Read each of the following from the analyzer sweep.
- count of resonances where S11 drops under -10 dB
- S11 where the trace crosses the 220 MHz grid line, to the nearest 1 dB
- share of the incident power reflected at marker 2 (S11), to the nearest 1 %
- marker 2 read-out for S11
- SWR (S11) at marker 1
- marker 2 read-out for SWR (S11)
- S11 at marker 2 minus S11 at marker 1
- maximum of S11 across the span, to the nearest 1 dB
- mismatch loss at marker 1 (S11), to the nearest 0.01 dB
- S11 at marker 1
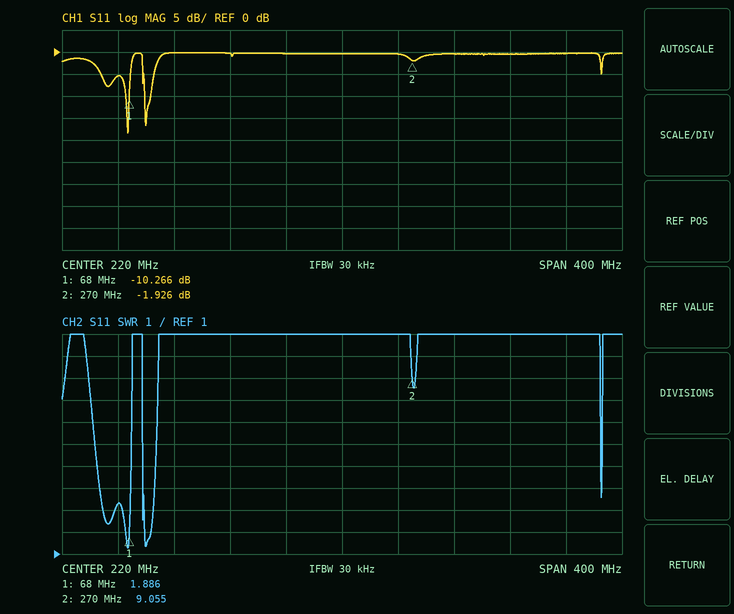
2
0 dB
64 %
-1.926 dB
1.886
9.055
8.340 dB
0 dB
0.43 dB
-10.266 dB
